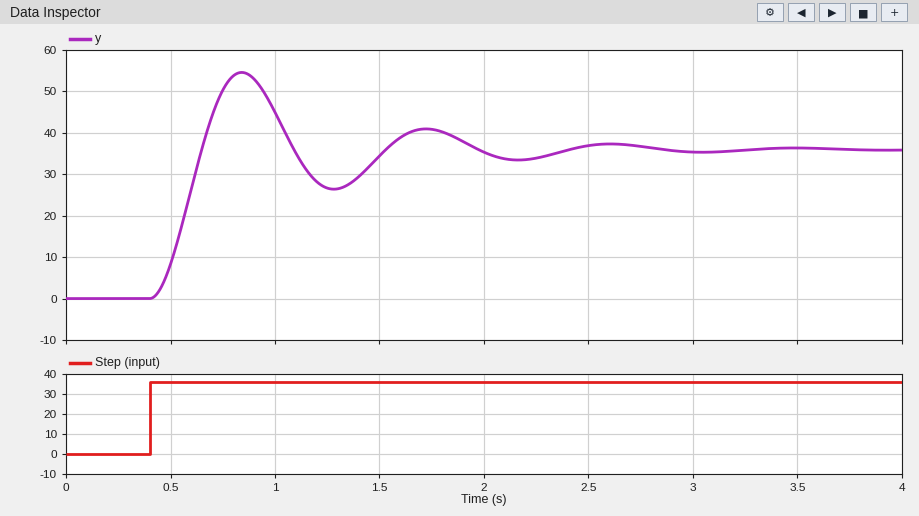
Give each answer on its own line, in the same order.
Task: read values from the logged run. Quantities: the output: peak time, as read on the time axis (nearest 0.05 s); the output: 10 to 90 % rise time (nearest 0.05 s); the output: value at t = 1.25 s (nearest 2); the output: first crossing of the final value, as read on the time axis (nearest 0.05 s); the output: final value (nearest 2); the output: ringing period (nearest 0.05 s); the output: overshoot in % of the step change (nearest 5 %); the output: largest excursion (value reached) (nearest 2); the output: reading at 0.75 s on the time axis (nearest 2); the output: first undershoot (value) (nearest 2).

0.85 s
0.15 s
26
0.65 s
36
0.90 s
50 %
54
50
26
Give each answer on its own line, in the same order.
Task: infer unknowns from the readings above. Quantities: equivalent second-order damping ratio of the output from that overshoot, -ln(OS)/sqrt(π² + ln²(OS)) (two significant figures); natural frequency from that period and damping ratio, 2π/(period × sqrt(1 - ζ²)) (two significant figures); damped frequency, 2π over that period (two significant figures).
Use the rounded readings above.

0.22
7.2 rad/s
7.0 rad/s
